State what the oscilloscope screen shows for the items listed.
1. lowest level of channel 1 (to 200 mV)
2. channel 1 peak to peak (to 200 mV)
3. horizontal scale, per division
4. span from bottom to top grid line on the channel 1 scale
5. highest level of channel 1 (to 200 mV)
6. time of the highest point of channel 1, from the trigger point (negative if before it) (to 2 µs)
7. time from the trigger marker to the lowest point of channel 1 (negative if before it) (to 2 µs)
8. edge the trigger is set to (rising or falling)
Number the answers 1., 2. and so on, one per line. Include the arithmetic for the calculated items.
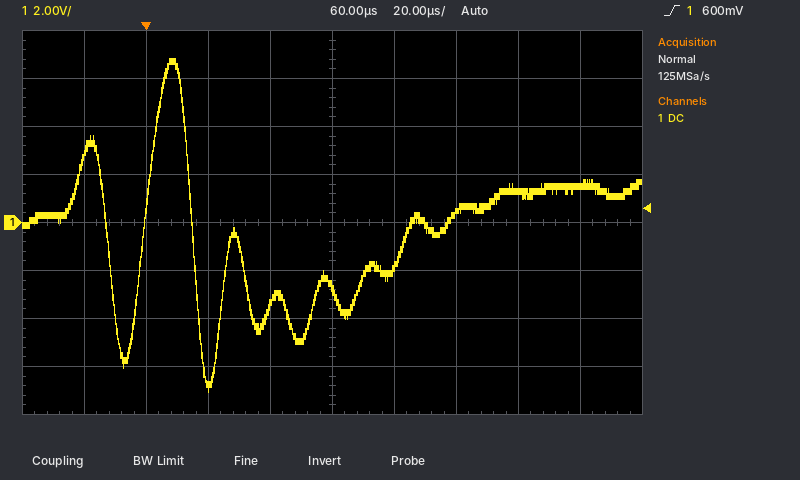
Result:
1. -7.0 V
2. 6.8 V − (-7.0 V) = 13.8 V
3. 20 µs
4. 16 V
5. 6.8 V
6. +8 µs
7. +20 µs
8. rising
